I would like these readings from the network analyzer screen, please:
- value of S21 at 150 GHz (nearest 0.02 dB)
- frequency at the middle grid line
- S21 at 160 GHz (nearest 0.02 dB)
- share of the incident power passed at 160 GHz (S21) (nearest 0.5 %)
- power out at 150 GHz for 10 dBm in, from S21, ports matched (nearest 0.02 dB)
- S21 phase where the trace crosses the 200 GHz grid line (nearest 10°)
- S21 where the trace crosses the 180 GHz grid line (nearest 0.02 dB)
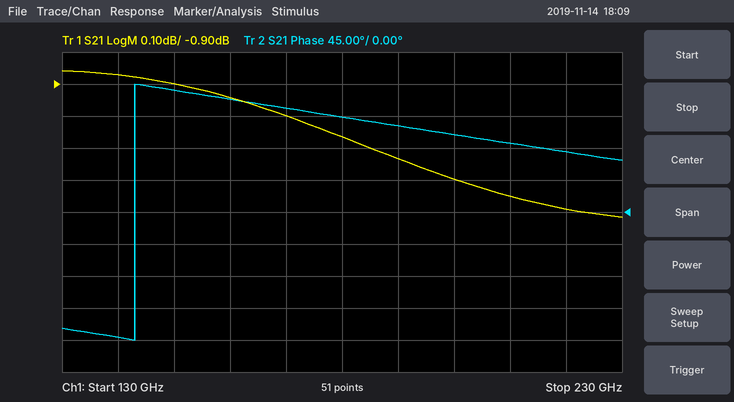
-0.90 dB
180 GHz
-0.94 dB
80.5 %
9.10 dBm
110°
-1.06 dB
